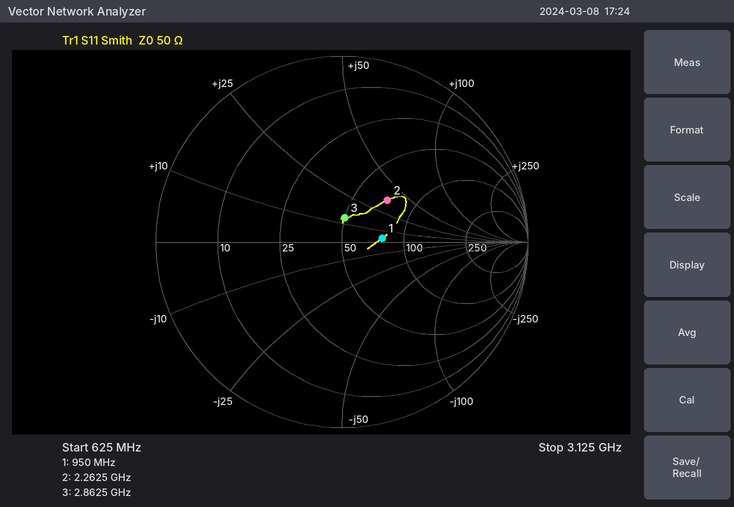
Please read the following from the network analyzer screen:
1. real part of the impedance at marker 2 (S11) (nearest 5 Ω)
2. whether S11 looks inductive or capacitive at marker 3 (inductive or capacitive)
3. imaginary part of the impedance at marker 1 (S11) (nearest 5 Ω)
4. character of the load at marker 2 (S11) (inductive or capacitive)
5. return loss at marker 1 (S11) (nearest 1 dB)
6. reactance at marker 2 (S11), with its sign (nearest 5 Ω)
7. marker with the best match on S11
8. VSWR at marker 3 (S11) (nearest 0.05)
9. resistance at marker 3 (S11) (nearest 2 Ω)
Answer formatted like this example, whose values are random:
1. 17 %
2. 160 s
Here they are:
1. 70 Ω
2. inductive
3. +5 Ω
4. inductive
5. 13 dB
6. +35 Ω
7. marker 3
8. 1.30
9. 50 Ω
